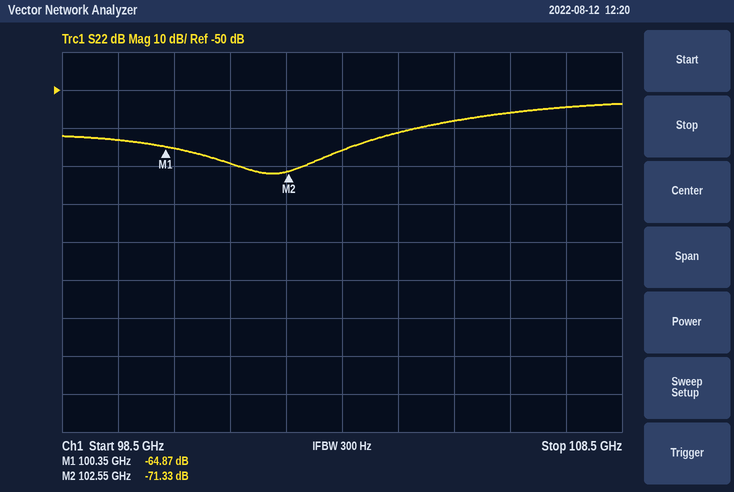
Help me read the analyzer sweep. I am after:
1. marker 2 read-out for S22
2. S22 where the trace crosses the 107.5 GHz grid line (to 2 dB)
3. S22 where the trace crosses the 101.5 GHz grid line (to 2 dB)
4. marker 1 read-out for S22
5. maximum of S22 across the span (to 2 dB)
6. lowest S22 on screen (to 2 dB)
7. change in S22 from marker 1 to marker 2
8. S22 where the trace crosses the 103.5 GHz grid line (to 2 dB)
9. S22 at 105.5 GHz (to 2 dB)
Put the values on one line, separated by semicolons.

-71.33 dB; -54 dB; -70 dB; -64.87 dB; -54 dB; -72 dB; -6.46 dB; -66 dB; -58 dB
